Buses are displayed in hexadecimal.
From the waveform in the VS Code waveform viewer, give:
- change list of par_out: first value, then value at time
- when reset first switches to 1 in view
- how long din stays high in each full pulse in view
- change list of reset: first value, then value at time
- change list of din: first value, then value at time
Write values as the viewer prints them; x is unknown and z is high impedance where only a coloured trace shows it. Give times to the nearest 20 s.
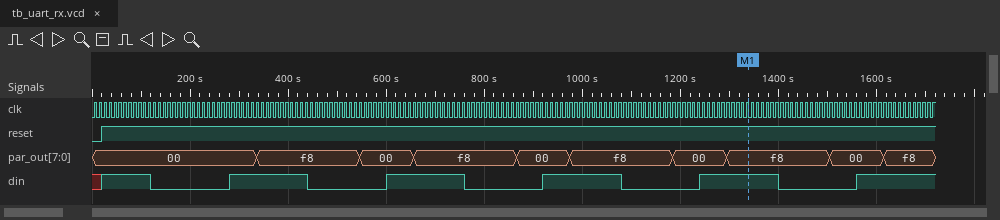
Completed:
00, f8 at 340 s, 00 at 540 s, f8 at 660 s, 00 at 860 s, f8 at 980 s, 00 at 1180 s, f8 at 1300 s, 00 at 1500 s, f8 at 1620 s
20 s
160 s, 160 s, 160 s, 160 s
0, 1 at 20 s
x, 1 at 20 s, 0 at 120 s, 1 at 280 s, 0 at 440 s, 1 at 600 s, 0 at 760 s, 1 at 920 s, 0 at 1080 s, 1 at 1240 s, 0 at 1400 s, 1 at 1560 s
